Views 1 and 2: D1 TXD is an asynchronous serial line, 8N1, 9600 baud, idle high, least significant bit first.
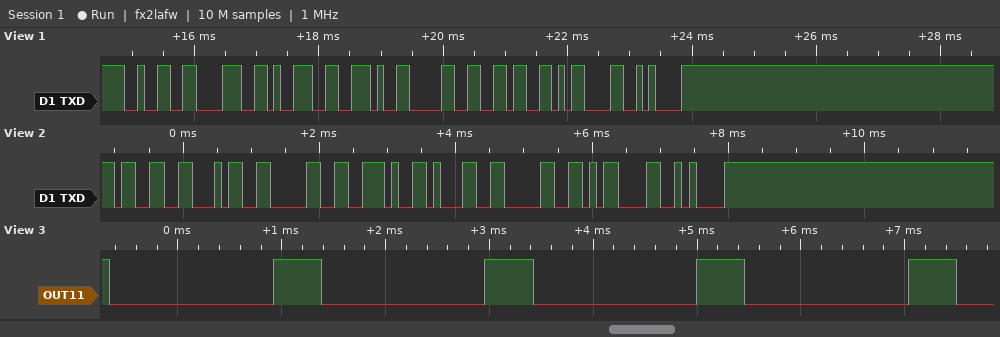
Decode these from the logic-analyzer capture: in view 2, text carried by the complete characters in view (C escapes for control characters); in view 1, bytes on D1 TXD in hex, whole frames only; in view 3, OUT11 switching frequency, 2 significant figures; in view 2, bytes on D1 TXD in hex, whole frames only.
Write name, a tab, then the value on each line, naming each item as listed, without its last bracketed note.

in view 2, text carried by the complete characters in view	"340.10\r\n"
in view 1, bytes on D1 TXD in hex, whole frames only	32 38 39 2E 30 36 0D 0A
in view 3, OUT11 switching frequency, 2 significant figures	490 Hz
in view 2, bytes on D1 TXD in hex, whole frames only	33 34 30 2E 31 30 0D 0A
